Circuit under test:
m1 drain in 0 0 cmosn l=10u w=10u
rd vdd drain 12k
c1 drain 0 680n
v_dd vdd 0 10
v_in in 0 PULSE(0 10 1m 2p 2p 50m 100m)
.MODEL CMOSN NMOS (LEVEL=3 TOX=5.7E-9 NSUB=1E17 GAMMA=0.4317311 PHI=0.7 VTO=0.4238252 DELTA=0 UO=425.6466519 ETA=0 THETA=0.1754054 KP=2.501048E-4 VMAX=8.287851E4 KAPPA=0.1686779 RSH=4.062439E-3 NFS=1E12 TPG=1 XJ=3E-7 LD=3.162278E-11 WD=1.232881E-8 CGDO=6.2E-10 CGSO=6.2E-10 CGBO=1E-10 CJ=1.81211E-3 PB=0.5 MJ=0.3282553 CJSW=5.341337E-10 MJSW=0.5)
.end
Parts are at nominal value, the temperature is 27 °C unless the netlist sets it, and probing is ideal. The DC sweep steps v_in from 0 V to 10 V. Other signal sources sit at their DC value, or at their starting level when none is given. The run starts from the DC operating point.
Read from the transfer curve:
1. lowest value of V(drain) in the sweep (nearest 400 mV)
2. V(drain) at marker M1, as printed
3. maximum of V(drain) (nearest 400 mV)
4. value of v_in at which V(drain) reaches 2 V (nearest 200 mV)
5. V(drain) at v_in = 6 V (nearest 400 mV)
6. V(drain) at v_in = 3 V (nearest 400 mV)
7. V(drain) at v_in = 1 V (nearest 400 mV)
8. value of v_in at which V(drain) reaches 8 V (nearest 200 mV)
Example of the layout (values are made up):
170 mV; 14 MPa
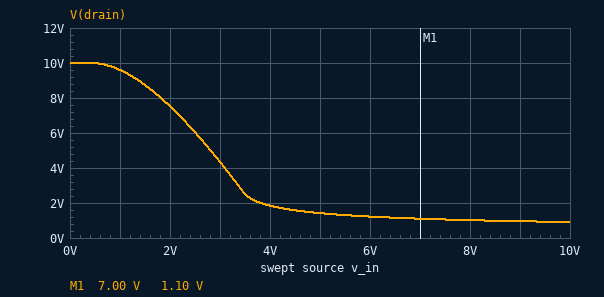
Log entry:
800 mV; 1.10 V; 10.0 V; 3.8 V; 1.2 V; 4.4 V; 9.6 V; 1.8 V
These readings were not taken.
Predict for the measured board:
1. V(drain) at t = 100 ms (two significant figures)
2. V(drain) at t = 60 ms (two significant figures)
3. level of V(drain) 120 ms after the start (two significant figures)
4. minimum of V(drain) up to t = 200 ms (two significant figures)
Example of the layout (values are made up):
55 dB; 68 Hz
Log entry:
10 V; 7.0 V; 910 mV; 910 mV
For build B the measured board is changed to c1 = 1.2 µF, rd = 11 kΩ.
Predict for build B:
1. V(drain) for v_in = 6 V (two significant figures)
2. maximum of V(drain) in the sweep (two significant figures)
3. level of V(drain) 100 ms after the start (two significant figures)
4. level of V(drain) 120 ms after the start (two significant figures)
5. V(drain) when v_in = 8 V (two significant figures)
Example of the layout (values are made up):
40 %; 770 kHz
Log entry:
1.3 V; 10 V; 9.8 V; 990 mV; 1.1 V
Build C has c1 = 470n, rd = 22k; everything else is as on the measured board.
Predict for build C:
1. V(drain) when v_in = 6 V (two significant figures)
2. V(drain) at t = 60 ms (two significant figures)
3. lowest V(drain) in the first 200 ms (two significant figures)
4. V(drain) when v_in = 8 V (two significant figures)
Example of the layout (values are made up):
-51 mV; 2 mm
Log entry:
660 mV; 6.0 V; 500 mV; 560 mV
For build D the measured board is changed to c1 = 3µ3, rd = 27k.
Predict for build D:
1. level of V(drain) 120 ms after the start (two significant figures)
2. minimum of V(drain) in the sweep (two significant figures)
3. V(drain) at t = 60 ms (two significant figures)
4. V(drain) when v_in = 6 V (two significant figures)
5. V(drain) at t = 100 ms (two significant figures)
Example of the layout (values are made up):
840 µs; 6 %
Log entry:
450 mV; 410 mV; 1.3 V; 530 mV; 4.5 V
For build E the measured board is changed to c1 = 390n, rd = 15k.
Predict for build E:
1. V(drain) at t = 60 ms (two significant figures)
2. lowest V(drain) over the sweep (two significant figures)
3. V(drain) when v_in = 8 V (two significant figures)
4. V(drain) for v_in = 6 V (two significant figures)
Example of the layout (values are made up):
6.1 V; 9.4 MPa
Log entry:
8.0 V; 730 mV; 820 mV; 970 mV
